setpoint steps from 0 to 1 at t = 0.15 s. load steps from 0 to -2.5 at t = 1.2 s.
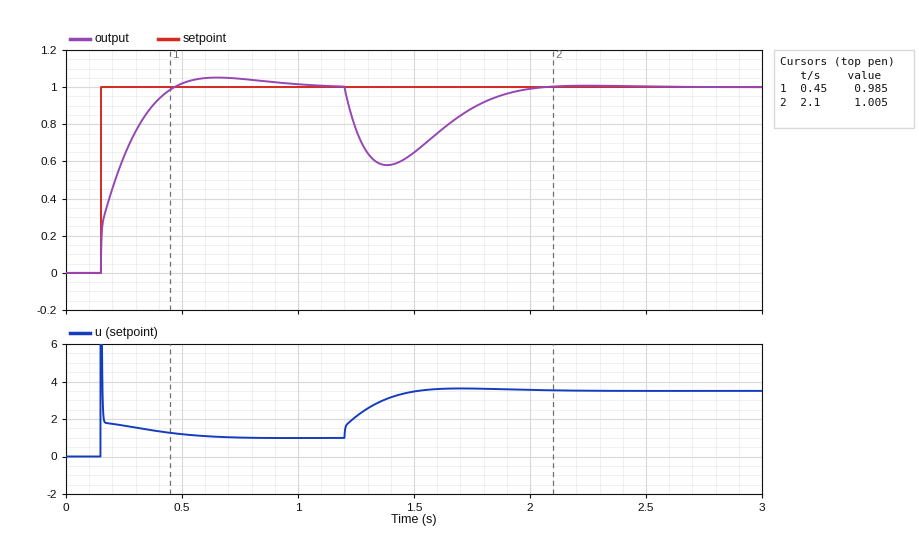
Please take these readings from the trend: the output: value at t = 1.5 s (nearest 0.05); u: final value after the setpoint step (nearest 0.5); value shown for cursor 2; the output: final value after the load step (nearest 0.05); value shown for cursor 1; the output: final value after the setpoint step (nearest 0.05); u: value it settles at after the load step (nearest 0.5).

0.65
1.0
1.005
1.00
0.985
1.00
3.5
